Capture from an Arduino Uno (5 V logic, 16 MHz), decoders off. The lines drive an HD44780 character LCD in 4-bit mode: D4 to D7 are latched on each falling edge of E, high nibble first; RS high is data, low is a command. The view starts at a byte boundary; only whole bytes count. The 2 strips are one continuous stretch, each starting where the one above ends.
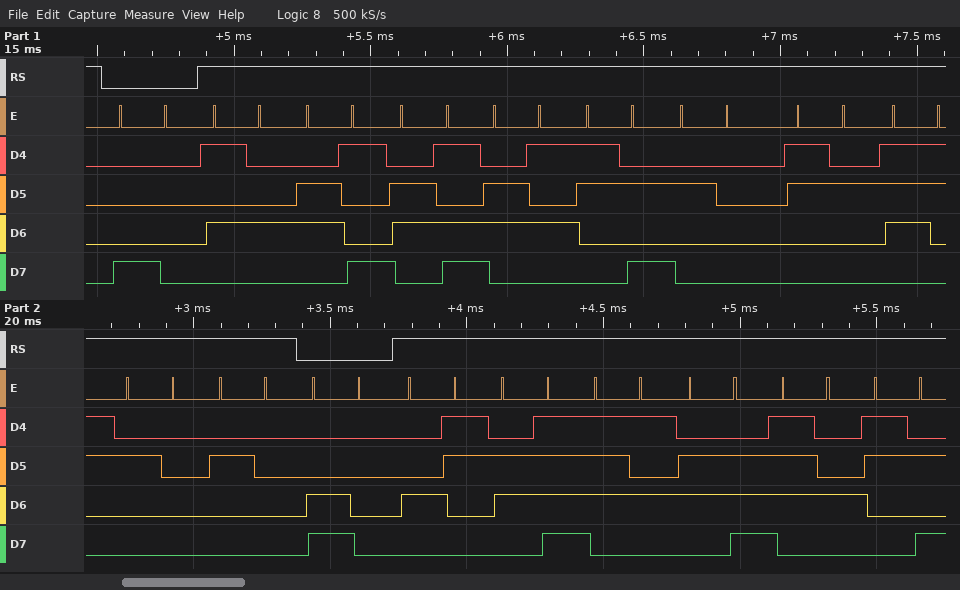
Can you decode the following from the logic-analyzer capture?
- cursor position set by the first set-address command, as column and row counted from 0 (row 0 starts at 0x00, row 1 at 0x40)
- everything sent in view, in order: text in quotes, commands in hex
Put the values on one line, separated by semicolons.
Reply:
column 0, row 0; 0x80 "Time: 2s  " 0xC0 "Count:"
